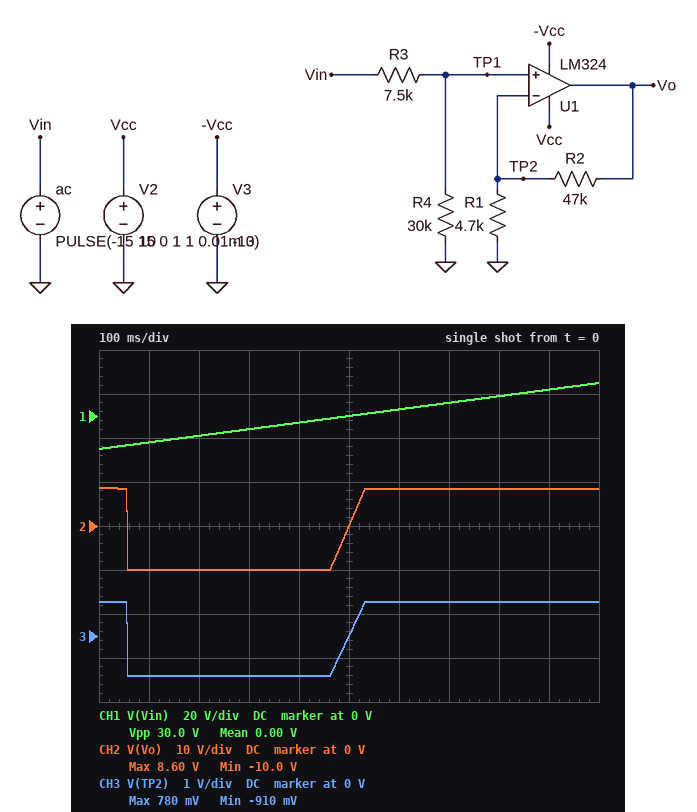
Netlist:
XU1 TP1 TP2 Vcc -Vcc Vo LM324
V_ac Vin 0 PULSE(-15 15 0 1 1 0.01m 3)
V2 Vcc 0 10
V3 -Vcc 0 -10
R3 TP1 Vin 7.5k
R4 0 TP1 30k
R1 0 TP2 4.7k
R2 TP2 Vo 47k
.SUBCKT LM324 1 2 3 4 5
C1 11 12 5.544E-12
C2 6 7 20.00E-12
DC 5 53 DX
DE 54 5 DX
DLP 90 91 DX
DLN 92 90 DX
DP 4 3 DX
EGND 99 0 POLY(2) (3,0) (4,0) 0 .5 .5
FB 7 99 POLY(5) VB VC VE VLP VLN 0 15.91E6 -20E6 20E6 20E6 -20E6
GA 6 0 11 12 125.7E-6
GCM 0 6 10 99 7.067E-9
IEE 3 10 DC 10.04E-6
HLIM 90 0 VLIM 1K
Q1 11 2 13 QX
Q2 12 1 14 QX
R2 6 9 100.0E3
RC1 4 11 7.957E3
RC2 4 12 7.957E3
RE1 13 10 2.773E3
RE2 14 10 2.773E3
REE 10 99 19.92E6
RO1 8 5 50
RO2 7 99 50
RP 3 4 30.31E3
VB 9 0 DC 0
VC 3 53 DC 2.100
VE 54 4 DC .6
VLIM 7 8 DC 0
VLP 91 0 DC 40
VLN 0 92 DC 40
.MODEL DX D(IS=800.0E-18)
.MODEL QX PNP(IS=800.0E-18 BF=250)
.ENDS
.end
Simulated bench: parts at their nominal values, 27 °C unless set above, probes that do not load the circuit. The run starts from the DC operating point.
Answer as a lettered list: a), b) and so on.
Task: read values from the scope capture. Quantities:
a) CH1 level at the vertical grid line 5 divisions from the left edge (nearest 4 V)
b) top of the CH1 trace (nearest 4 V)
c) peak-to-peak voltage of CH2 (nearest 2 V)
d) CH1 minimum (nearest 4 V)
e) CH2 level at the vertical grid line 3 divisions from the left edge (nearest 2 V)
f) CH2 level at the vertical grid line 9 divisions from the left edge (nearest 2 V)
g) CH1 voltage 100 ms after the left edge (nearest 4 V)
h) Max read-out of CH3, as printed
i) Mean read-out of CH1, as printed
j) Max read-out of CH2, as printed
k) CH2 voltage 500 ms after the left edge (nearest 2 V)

a) 0 V
b) 16 V
c) 18 V
d) -16 V
e) -10 V
f) 8 V
g) -12 V
h) 780 mV
i) 0.00 V
j) 8.60 V
k) 0 V
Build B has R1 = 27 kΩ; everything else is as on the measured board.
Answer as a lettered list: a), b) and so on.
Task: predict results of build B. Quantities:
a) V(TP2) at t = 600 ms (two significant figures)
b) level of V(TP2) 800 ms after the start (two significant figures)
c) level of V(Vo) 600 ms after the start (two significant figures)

a) 2.4 V
b) 3.1 V
c) 6.6 V
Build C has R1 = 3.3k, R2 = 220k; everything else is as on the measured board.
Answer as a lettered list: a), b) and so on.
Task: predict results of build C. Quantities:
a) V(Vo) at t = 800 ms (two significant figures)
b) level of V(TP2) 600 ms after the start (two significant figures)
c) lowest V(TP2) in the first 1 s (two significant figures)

a) 8.5 V
b) 130 mV
c) -150 mV
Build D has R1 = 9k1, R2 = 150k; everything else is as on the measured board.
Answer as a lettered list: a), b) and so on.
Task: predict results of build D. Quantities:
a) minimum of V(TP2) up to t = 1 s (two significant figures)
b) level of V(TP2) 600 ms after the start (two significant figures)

a) -570 mV
b) 490 mV
